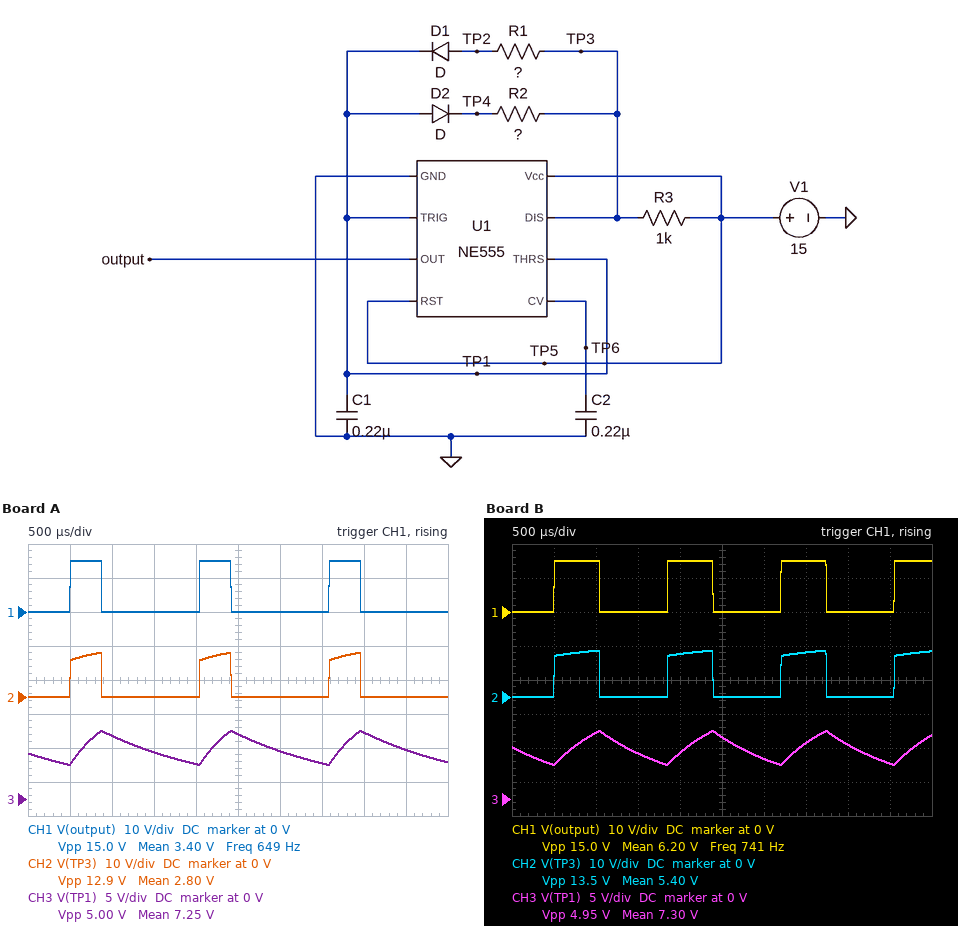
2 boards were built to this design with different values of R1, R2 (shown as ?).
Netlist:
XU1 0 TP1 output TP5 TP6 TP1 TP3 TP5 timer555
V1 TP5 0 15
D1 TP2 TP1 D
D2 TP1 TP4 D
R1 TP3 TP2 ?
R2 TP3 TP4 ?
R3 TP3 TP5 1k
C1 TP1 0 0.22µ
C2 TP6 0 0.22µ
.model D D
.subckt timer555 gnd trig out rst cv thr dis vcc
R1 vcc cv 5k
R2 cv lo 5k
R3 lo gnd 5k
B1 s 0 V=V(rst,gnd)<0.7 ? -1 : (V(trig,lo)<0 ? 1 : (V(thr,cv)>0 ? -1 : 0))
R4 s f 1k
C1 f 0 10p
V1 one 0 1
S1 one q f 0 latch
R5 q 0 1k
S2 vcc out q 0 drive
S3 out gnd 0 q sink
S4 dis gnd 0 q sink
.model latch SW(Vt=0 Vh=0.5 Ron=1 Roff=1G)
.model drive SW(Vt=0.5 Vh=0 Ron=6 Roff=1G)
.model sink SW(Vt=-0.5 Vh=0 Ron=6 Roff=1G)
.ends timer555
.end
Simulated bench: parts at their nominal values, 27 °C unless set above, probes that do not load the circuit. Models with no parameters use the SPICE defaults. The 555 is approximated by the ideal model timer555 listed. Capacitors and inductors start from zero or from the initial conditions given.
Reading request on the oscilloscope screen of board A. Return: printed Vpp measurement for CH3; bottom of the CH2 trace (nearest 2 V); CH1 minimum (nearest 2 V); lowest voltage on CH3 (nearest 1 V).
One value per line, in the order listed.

5.00 V
0 V
0 V
5 V
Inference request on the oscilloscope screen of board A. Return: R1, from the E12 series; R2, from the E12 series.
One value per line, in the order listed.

1.2 kΩ
6.8 kΩ
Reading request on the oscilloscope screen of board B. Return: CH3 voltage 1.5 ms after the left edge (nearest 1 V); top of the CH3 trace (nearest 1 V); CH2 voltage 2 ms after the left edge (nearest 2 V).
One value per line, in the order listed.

7 V
10 V
12 V
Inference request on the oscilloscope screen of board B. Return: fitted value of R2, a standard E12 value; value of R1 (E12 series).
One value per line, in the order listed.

4.7 kΩ
2.2 kΩ
